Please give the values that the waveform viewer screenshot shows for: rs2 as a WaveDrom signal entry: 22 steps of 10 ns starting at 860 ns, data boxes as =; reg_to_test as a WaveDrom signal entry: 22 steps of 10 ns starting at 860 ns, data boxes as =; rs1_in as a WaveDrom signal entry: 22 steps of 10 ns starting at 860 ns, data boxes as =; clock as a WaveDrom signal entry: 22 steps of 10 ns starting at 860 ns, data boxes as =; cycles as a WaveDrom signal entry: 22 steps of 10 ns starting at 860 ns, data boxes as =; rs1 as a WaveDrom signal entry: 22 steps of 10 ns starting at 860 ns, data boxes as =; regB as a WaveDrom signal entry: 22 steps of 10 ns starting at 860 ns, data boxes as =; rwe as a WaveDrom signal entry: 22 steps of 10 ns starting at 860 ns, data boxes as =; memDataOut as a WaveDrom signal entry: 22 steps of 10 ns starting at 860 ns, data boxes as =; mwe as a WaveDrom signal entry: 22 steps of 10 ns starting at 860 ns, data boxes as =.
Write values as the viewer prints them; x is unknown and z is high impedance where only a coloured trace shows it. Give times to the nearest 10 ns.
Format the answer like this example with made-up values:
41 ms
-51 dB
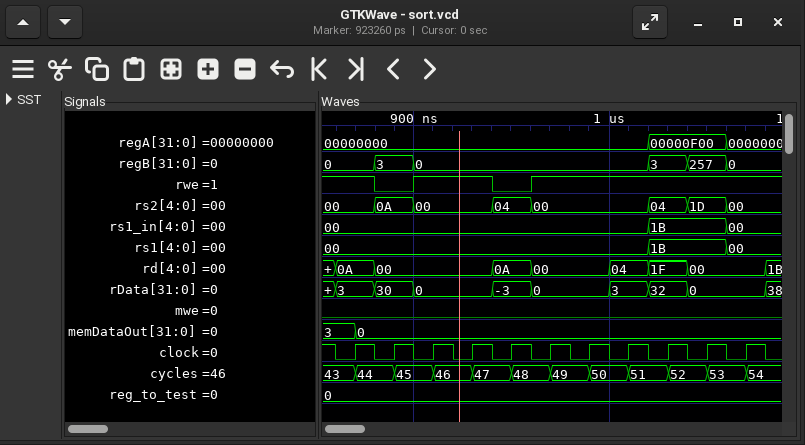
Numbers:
{name: 'rs2', wave: '=.=.=...=.=.....=.=.=.', data: '00 0A 00 04 00 04 1D 00'}
{name: 'reg_to_test', wave: '=.....................', data: '0'}
{name: 'rs1_in', wave: '=...............=...=.', data: '00 1B 00'}
{name: 'clock', wave: '0101010101010101010101'}
{name: 'cycles', wave: '==.=.=.=.=.=.=.=.=.=.=', data: '43 44 45 46 47 48 49 50 51 52 53 54'}
{name: 'rs1', wave: '=...............=...=.', data: '00 1B 00'}
{name: 'regB', wave: '=.=.=...........=.=.=.', data: '0 3 0 3 257 0'}
{name: 'rwe', wave: '1.0.1...0.1...........'}
{name: 'memDataOut', wave: '==....................', data: '3 0'}
{name: 'mwe', wave: '0.....................'}
